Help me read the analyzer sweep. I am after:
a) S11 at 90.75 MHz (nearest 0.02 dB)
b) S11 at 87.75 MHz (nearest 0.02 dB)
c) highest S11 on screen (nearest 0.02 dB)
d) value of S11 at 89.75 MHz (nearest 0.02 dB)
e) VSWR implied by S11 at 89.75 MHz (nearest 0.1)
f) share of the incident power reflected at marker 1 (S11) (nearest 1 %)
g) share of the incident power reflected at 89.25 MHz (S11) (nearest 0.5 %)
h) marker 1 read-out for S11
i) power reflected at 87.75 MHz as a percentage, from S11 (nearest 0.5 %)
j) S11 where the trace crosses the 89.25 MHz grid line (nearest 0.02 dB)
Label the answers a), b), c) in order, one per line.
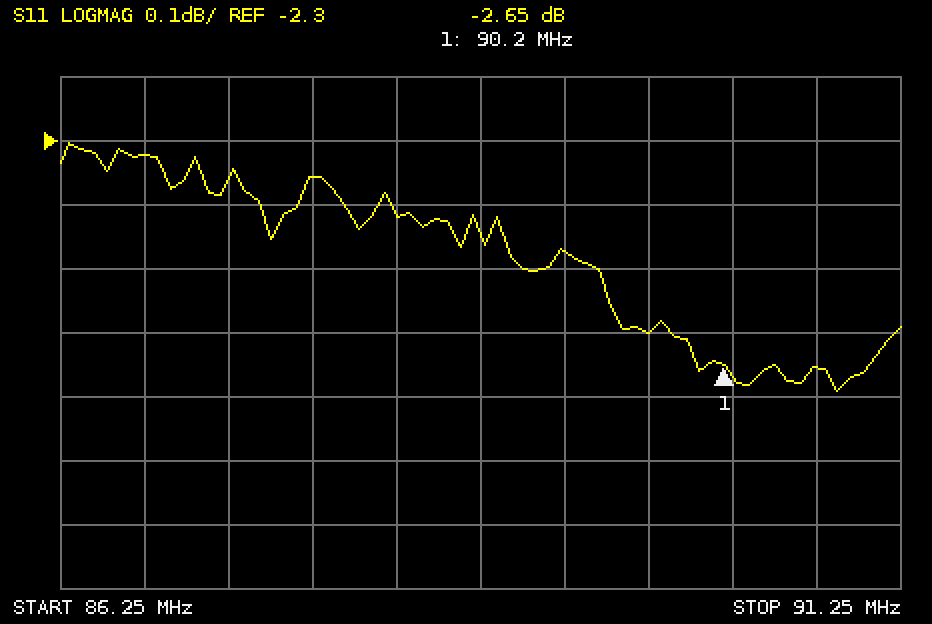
a) -2.66 dB
b) -2.36 dB
c) -2.30 dB
d) -2.60 dB
e) 6.7
f) 54 %
g) 56.5 %
h) -2.65 dB
i) 58.0 %
j) -2.48 dB
